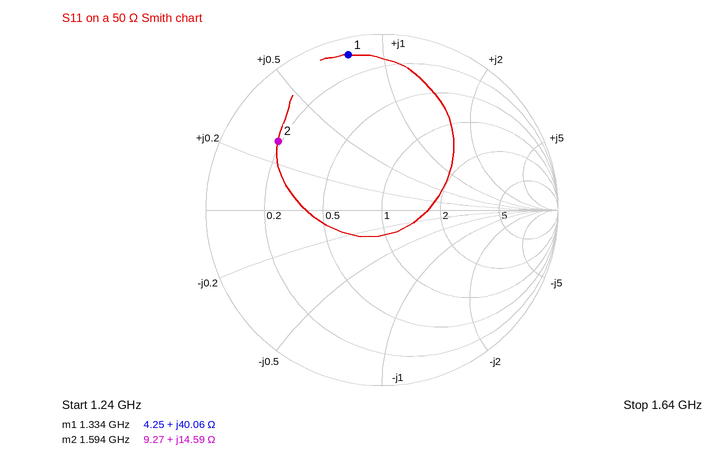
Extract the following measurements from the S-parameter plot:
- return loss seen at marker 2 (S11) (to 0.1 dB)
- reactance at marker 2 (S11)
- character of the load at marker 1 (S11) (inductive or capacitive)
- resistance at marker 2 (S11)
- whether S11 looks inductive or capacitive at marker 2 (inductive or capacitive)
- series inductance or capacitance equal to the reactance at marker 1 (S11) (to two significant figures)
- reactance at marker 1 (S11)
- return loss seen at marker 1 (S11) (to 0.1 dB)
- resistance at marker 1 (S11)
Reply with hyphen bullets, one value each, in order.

- 3.0 dB
- +14.59 Ω
- inductive
- 9.27 Ω
- inductive
- 4.8 nH
- +40.06 Ω
- 0.9 dB
- 4.25 Ω
